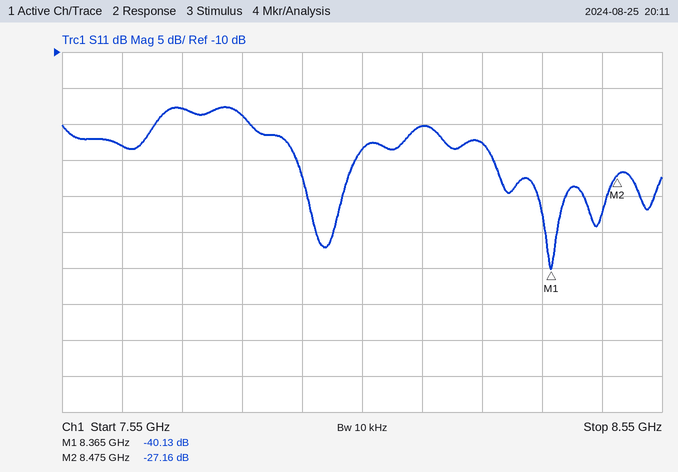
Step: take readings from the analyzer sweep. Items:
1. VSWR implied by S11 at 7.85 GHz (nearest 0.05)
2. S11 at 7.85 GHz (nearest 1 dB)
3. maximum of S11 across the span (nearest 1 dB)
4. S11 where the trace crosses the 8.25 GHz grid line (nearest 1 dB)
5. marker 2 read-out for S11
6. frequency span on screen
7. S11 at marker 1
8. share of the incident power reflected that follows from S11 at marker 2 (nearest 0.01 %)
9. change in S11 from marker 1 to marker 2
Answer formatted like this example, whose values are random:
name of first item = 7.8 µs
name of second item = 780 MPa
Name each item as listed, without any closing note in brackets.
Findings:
VSWR implied by S11 at 7.85 GHz = 1.25
S11 at 7.85 GHz = -19 dB
maximum of S11 across the span = -18 dB
S11 where the trace crosses the 8.25 GHz grid line = -23 dB
marker 2 read-out for S11 = -27.16 dB
frequency span on screen = 1 GHz
S11 at marker 1 = -40.13 dB
share of the incident power reflected that follows from S11 at marker 2 = 0.19 %
change in S11 from marker 1 to marker 2 = 12.97 dB
